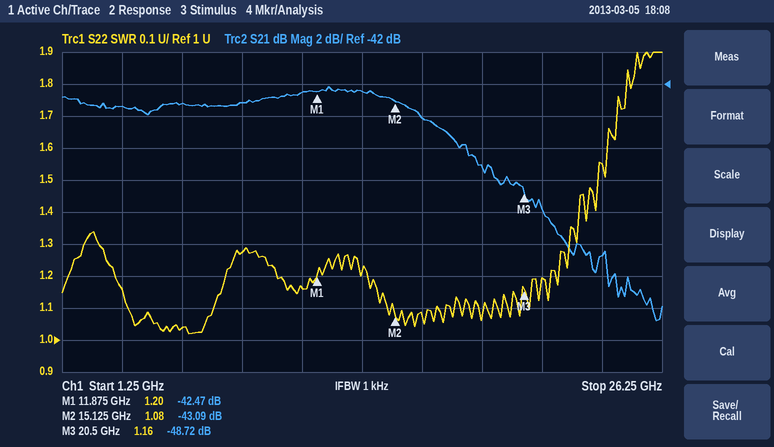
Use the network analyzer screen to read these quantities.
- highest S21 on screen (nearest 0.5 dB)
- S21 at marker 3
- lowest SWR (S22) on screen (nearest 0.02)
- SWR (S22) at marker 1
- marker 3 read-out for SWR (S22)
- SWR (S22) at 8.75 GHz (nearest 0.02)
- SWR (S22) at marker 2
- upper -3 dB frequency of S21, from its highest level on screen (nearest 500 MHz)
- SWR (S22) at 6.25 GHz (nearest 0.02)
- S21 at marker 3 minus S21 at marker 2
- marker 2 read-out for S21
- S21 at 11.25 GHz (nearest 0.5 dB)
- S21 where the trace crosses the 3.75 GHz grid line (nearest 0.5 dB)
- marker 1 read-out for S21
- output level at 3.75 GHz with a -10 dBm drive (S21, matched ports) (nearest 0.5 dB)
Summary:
-42.0 dB
-48.72 dB
1.02
1.20
1.16
1.28
1.08
17.5 GHz
1.04
-5.63 dB
-43.09 dB
-42.5 dB
-43.5 dB
-42.47 dB
-53.5 dBm
